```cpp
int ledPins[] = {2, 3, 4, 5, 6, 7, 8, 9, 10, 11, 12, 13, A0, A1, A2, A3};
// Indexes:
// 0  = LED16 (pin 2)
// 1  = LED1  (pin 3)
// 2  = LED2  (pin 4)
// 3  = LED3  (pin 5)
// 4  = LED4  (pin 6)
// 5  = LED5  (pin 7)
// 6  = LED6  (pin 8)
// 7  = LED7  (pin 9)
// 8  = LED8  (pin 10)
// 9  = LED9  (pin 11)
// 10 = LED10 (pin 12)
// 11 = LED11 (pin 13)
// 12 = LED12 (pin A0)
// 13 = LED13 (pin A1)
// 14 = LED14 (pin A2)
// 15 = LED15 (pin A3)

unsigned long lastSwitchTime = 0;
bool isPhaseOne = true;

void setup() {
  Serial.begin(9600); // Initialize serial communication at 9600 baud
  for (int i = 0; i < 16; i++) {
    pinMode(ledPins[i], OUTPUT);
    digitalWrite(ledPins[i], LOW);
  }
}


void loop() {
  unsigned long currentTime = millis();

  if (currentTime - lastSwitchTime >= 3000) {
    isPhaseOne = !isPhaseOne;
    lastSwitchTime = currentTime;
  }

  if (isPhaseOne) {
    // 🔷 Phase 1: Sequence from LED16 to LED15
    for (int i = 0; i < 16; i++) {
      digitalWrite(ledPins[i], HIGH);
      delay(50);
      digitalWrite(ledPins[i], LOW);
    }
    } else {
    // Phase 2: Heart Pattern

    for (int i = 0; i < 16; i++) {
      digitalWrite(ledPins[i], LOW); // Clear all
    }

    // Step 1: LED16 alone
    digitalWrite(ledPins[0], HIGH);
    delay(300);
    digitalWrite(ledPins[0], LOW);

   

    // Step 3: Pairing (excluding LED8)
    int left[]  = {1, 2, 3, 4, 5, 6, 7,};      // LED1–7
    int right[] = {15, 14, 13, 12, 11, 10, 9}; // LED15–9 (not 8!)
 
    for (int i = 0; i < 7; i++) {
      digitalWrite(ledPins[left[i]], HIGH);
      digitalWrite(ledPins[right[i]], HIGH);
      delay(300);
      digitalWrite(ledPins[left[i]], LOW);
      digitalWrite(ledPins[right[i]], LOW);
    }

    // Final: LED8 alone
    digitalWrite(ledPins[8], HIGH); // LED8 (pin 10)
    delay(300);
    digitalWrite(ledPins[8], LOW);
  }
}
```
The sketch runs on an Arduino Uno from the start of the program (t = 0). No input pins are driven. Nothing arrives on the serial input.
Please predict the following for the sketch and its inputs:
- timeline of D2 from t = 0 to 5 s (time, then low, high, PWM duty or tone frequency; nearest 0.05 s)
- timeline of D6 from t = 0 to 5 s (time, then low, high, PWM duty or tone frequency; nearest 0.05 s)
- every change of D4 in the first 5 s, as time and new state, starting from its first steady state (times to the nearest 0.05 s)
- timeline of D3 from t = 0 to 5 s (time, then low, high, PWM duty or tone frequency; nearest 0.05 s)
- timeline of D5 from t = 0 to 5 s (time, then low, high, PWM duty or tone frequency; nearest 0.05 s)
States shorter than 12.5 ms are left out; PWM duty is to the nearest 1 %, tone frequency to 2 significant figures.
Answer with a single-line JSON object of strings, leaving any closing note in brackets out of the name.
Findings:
{"timeline of D2 from t = 0 to 5 s": "0 s high; 0.05 s low; 0.8 s high; 0.85 s low; 1.6 s high; 1.65 s low; 2.4 s high; 2.45 s low; 3.2 s high; 3.5 s low", "timeline of D6 from t = 0 to 5 s": "0 s low; 0.2 s high; 0.25 s low; 1 s high; 1.05 s low; 1.8 s high; 1.85 s low; 2.6 s high; 2.65 s low; 4.4 s high; 4.7 s low", "every change of D4 in the first 5 s, as time and new state, starting from its first steady state": "0 s low; 0.1 s high; 0.15 s low; 0.9 s high; 0.95 s low; 1.7 s high; 1.75 s low; 2.5 s high; 2.55 s low; 3.8 s high; 4.1 s low", "timeline of D3 from t = 0 to 5 s": "0 s low; 0.05 s high; 0.1 s low; 0.85 s high; 0.9 s low; 1.65 s high; 1.7 s low; 2.45 s high; 2.5 s low; 3.5 s high; 3.8 s low", "timeline of D5 from t = 0 to 5 s": "0 s low; 0.15 s high; 0.2 s low; 0.95 s high; 1 s low; 1.75 s high; 1.8 s low; 2.55 s high; 2.6 s low; 4.1 s high; 4.4 s low"}
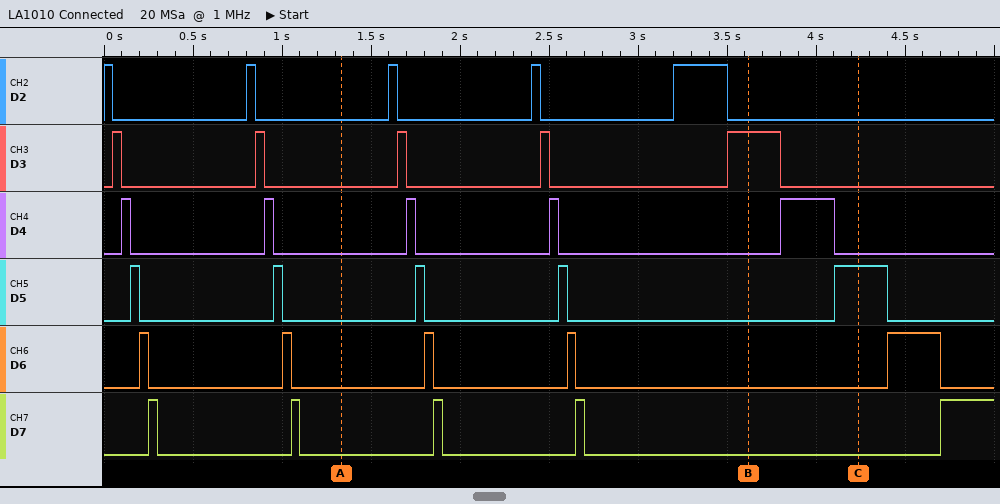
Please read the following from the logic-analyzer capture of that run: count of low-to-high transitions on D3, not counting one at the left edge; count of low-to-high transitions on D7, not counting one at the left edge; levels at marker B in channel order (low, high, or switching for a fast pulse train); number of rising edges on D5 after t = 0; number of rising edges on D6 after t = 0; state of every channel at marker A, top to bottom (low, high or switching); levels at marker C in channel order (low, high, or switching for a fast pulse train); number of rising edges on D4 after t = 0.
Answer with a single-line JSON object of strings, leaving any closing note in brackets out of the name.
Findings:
{"count of low-to-high transitions on D3, not counting one at the left edge": "5", "count of low-to-high transitions on D7, not counting one at the left edge": "5", "levels at marker B in channel order": "D2 low, D3 high, D4 low, D5 low, D6 low, D7 low", "number of rising edges on D5 after t = 0": "5", "number of rising edges on D6 after t = 0": "5", "state of every channel at marker A, top to bottom": "D2 low, D3 low, D4 low, D5 low, D6 low, D7 low", "levels at marker C in channel order": "D2 low, D3 low, D4 low, D5 high, D6 low, D7 low", "number of rising edges on D4 after t = 0": "5"}
